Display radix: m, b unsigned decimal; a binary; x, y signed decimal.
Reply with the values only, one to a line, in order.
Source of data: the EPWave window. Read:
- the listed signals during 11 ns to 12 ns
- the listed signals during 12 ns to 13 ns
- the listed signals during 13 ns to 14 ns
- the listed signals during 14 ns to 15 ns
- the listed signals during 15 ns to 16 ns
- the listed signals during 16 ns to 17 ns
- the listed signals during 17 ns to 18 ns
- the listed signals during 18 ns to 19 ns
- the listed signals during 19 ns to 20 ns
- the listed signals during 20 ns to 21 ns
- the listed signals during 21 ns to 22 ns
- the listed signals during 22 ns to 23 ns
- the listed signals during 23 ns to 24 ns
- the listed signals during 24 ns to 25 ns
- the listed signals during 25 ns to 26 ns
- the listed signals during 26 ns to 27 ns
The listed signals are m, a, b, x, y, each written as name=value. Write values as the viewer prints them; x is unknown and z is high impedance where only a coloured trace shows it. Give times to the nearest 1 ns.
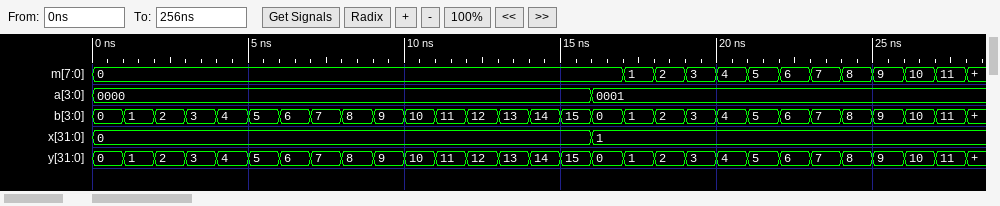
m=0, a=0000, b=11, x=0, y=11
m=0, a=0000, b=12, x=0, y=12
m=0, a=0000, b=13, x=0, y=13
m=0, a=0000, b=14, x=0, y=14
m=0, a=0000, b=15, x=0, y=15
m=0, a=0001, b=0, x=1, y=0
m=1, a=0001, b=1, x=1, y=1
m=2, a=0001, b=2, x=1, y=2
m=3, a=0001, b=3, x=1, y=3
m=4, a=0001, b=4, x=1, y=4
m=5, a=0001, b=5, x=1, y=5
m=6, a=0001, b=6, x=1, y=6
m=7, a=0001, b=7, x=1, y=7
m=8, a=0001, b=8, x=1, y=8
m=9, a=0001, b=9, x=1, y=9
m=10, a=0001, b=10, x=1, y=10
